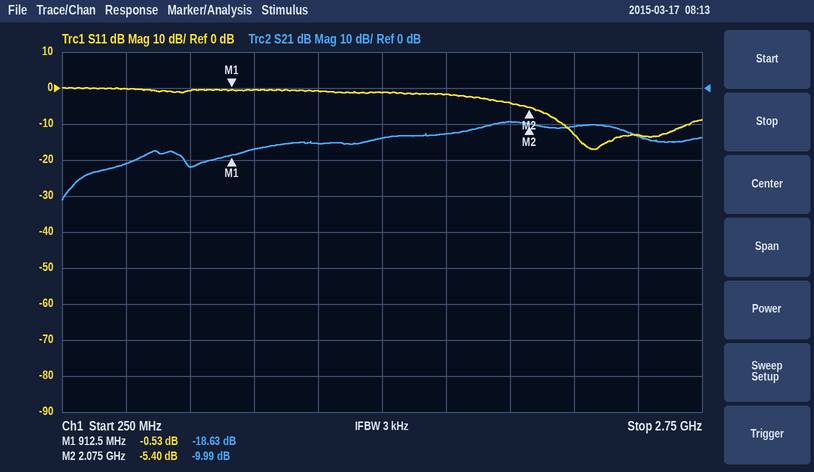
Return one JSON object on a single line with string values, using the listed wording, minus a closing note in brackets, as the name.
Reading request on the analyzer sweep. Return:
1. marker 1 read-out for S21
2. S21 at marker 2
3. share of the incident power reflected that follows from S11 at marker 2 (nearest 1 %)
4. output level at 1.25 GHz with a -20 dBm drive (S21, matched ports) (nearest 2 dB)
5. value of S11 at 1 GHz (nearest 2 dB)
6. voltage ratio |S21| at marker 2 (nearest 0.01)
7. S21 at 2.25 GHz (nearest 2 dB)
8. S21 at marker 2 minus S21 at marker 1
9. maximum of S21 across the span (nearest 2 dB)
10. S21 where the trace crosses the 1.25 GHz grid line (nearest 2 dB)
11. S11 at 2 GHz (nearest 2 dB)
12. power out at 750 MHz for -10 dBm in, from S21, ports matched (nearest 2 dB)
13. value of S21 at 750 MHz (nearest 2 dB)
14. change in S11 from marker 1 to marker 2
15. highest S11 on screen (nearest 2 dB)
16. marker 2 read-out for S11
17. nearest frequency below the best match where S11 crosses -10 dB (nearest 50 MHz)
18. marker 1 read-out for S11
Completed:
{"marker 1 read-out for S21": "-18.63 dB", "S21 at marker 2": "-9.99 dB", "share of the incident power reflected that follows from S11 at marker 2": "29 %", "output level at 1.25 GHz with a -20 dBm drive (S21, matched ports)": "-36 dBm", "value of S11 at 1 GHz": "0 dB", "voltage ratio |S21| at marker 2": "0.32", "S21 at 2.25 GHz": "-10 dB", "S21 at marker 2 minus S21 at marker 1": "8.64 dB", "maximum of S21 across the span": "-10 dB", "S21 where the trace crosses the 1.25 GHz grid line": "-16 dB", "S11 at 2 GHz": "-4 dB", "power out at 750 MHz for -10 dBm in, from S21, ports matched": "-32 dBm", "value of S21 at 750 MHz": "-22 dB", "change in S11 from marker 1 to marker 2": "-4.87 dB", "highest S11 on screen": "0 dB", "marker 2 read-out for S11": "-5.40 dB", "nearest frequency below the best match where S11 crosses -10 dB": "2.20 GHz", "marker 1 read-out for S11": "-0.53 dB"}
